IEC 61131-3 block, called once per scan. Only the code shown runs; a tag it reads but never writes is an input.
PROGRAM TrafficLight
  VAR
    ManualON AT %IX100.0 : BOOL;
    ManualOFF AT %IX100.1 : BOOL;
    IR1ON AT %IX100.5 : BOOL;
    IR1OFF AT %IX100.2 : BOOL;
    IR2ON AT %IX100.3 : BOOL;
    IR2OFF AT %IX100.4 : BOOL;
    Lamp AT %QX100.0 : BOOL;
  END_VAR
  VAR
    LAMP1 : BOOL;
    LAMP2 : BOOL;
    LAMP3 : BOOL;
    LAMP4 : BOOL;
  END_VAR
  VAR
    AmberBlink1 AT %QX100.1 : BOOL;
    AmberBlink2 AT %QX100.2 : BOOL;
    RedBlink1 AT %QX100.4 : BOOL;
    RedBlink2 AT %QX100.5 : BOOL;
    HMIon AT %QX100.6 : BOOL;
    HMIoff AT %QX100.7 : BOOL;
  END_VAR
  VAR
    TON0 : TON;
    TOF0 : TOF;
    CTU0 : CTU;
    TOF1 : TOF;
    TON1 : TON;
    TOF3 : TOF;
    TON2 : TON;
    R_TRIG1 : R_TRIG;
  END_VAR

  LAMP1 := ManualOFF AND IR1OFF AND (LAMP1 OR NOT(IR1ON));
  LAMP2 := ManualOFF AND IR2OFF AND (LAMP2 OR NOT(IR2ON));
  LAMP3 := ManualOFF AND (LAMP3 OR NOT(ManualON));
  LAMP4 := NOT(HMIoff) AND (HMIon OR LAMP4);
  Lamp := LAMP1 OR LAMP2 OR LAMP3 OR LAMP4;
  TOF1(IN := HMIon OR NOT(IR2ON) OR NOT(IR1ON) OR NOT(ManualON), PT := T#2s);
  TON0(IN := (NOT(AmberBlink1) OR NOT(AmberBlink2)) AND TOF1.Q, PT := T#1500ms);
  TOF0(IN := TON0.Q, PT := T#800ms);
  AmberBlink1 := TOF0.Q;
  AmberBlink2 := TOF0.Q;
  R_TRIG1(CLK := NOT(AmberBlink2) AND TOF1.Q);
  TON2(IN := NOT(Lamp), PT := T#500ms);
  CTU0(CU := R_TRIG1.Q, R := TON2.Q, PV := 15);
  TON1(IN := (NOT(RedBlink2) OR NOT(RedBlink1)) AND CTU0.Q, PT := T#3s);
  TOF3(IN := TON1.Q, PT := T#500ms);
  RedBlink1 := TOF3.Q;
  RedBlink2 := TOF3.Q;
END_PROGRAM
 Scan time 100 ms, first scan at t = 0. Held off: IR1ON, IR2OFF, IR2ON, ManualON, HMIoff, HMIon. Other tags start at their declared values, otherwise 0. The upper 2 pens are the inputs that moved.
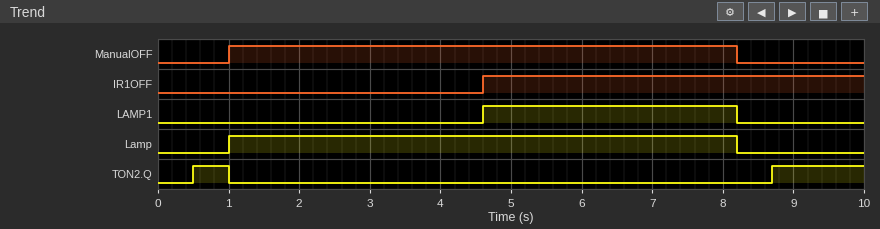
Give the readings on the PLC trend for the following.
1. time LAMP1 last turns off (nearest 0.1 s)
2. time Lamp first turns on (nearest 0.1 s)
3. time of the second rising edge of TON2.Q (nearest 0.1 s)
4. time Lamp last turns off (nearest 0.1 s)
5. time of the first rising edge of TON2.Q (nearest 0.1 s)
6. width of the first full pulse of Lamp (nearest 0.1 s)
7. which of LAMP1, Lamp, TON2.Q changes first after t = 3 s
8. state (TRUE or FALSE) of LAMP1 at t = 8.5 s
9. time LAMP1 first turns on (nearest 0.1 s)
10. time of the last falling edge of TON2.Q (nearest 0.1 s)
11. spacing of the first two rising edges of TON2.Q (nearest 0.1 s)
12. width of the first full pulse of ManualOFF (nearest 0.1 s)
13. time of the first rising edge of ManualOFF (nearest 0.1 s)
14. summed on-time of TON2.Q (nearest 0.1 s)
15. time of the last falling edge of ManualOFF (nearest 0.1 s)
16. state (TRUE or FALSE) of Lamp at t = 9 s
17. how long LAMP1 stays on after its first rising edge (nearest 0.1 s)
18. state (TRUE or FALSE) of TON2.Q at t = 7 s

8.2 s
1.0 s
8.7 s
8.2 s
0.5 s
7.2 s
LAMP1
FALSE
4.6 s
1.0 s
8.2 s
7.2 s
1.0 s
1.8 s
8.2 s
FALSE
3.6 s
FALSE
